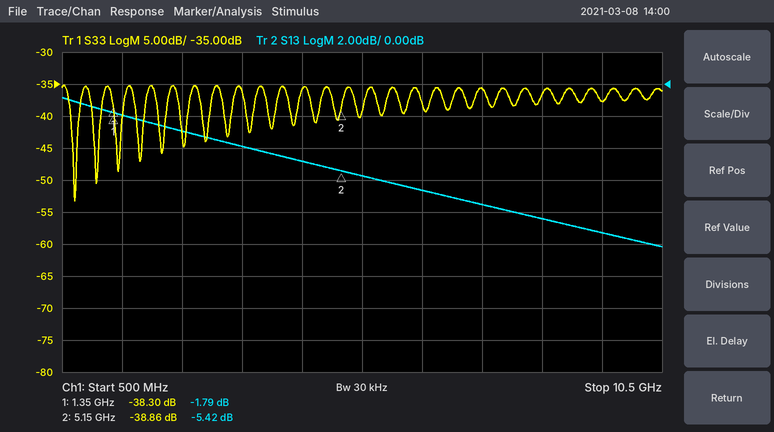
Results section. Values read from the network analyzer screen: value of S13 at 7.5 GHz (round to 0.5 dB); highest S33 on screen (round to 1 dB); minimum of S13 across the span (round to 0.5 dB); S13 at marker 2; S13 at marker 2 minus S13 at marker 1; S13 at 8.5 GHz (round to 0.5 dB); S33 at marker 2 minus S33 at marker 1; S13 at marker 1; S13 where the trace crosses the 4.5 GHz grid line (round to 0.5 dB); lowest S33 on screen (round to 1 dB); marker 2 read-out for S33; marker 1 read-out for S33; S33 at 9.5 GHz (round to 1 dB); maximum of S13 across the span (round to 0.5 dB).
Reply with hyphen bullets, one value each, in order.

- -7.5 dB
- -35 dB
- -10.0 dB
- -5.42 dB
- -3.63 dB
- -8.5 dB
- -0.56 dB
- -1.79 dB
- -5.0 dB
- -53 dB
- -38.86 dB
- -38.30 dB
- -38 dB
- -1.0 dB
